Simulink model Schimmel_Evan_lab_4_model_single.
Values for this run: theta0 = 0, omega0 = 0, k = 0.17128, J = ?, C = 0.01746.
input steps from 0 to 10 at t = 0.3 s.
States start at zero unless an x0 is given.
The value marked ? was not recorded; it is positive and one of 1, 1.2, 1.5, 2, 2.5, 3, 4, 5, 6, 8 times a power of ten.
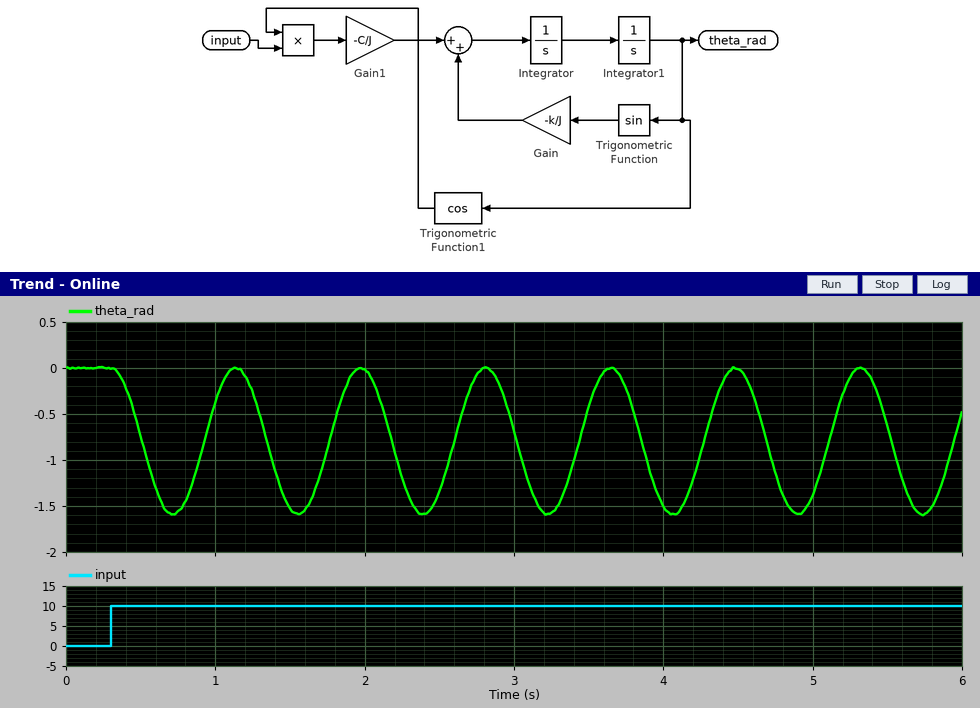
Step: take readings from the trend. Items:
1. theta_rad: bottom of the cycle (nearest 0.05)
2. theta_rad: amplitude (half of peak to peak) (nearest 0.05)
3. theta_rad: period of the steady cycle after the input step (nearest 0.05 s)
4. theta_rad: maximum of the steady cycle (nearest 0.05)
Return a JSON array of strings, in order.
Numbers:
["-1.60", "0.80", "0.85 s", "0.00"]
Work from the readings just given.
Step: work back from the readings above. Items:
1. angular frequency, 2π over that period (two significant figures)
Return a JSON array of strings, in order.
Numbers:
["7.4 rad/s"]
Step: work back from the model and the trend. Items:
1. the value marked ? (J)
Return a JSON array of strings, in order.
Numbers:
["0.004"]
